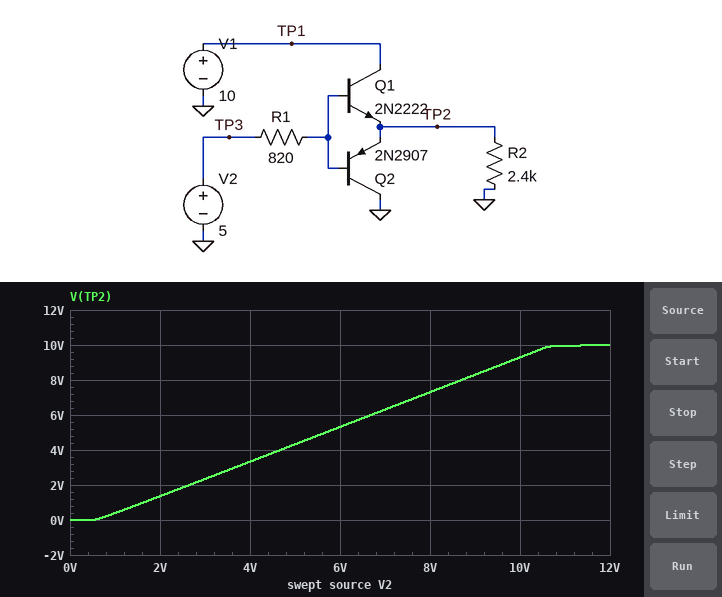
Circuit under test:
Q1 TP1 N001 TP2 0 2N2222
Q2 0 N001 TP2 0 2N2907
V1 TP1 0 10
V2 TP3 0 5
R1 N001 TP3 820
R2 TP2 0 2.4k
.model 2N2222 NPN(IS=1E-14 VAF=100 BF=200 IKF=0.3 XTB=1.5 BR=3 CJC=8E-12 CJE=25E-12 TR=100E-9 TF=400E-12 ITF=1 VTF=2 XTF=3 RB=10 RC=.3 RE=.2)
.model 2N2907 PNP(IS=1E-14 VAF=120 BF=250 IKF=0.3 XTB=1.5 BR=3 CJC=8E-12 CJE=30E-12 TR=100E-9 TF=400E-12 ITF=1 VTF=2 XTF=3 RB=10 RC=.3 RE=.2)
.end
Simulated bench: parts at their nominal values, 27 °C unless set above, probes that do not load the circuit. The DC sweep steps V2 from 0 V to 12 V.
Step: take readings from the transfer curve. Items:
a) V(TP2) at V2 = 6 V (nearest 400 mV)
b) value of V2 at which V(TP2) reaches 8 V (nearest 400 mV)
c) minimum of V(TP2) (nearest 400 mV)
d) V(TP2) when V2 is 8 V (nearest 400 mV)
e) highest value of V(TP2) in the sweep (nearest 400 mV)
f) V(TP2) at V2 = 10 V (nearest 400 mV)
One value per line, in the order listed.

5.2 V
8.8 V
0 V
7.2 V
10.0 V
9.2 V
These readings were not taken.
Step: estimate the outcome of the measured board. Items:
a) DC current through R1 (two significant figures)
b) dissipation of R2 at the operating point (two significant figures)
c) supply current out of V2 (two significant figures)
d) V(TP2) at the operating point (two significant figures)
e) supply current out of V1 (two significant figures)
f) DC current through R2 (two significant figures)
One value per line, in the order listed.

8.6 µA
7.8 mW
8.6 µA
4.3 V
1.8 mA
1.8 mA
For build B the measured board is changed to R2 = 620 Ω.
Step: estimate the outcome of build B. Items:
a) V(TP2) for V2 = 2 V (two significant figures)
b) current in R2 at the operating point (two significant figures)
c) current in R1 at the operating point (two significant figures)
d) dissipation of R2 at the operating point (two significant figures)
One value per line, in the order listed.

1.3 V
6.9 mA
33 µA
29 mW
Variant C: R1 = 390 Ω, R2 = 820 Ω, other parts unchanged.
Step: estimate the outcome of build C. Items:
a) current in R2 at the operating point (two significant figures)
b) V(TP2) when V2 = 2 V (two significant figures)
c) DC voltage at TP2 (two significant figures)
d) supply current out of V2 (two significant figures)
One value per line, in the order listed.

5.2 mA
1.3 V
4.3 V
25 µA
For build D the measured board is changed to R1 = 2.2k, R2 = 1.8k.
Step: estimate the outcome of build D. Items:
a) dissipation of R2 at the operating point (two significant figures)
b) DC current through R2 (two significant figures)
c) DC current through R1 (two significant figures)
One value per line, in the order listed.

10 mW
2.4 mA
11 µA
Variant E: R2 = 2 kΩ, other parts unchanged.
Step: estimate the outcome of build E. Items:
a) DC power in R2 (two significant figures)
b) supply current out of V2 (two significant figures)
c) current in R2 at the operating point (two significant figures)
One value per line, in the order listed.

9.3 mW
10 µA
2.2 mA
